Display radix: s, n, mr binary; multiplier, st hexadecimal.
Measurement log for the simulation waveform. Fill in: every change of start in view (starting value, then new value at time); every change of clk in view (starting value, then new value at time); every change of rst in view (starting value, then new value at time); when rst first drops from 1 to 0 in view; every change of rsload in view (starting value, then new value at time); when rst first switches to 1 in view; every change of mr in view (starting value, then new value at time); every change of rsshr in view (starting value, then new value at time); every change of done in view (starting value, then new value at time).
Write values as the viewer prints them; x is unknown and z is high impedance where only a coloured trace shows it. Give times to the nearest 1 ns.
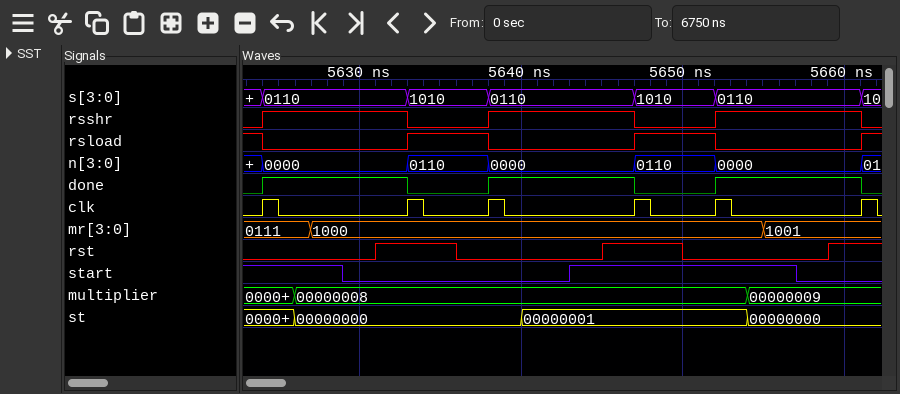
1, 0 at 5629 ns, 1 at 5643 ns, 0 at 5657 ns
0, 1 at 5624 ns, 0 at 5625 ns, 1 at 5633 ns, 0 at 5634 ns, 1 at 5638 ns, 0 at 5639 ns, 1 at 5647 ns, 0 at 5648 ns, 1 at 5652 ns, 0 at 5653 ns, 1 at 5661 ns, 0 at 5662 ns
0, 1 at 5631 ns, 0 at 5636 ns, 1 at 5645 ns, 0 at 5650 ns, 1 at 5659 ns
5636 ns
1, 0 at 5624 ns, 1 at 5633 ns, 0 at 5638 ns, 1 at 5647 ns, 0 at 5652 ns, 1 at 5661 ns
5631 ns
0111, 1000 at 5627 ns, 1001 at 5655 ns
0, 1 at 5624 ns, 0 at 5633 ns, 1 at 5638 ns, 0 at 5647 ns, 1 at 5652 ns, 0 at 5661 ns
0, 1 at 5624 ns, 0 at 5633 ns, 1 at 5638 ns, 0 at 5647 ns, 1 at 5652 ns, 0 at 5661 ns
